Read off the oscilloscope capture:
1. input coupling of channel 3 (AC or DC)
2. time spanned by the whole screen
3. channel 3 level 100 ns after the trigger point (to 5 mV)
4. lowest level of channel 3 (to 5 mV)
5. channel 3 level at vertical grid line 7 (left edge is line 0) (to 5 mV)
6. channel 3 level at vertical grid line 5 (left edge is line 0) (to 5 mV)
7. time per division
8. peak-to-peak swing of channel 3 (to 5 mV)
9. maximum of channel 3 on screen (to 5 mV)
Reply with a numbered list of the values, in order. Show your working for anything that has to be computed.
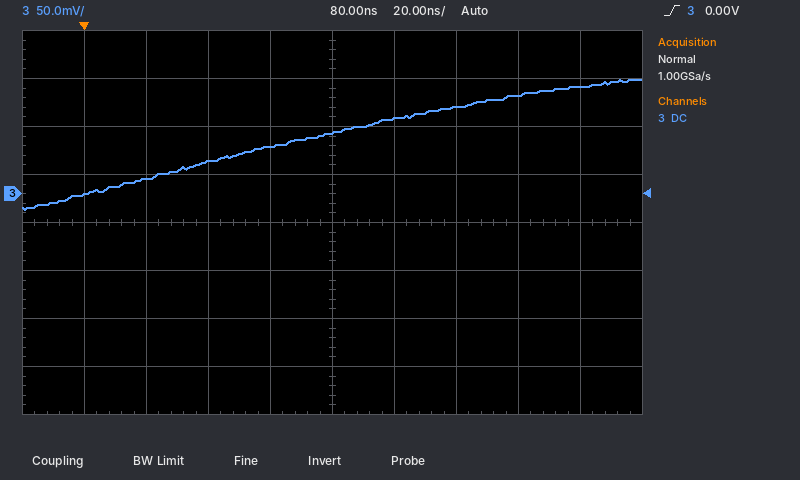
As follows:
1. DC
2. 200 ns
3. 80 mV
4. -15 mV
5. 90 mV
6. 65 mV
7. 20 ns
8. 120 mV − (-15 mV) = 135 mV
9. 120 mV
